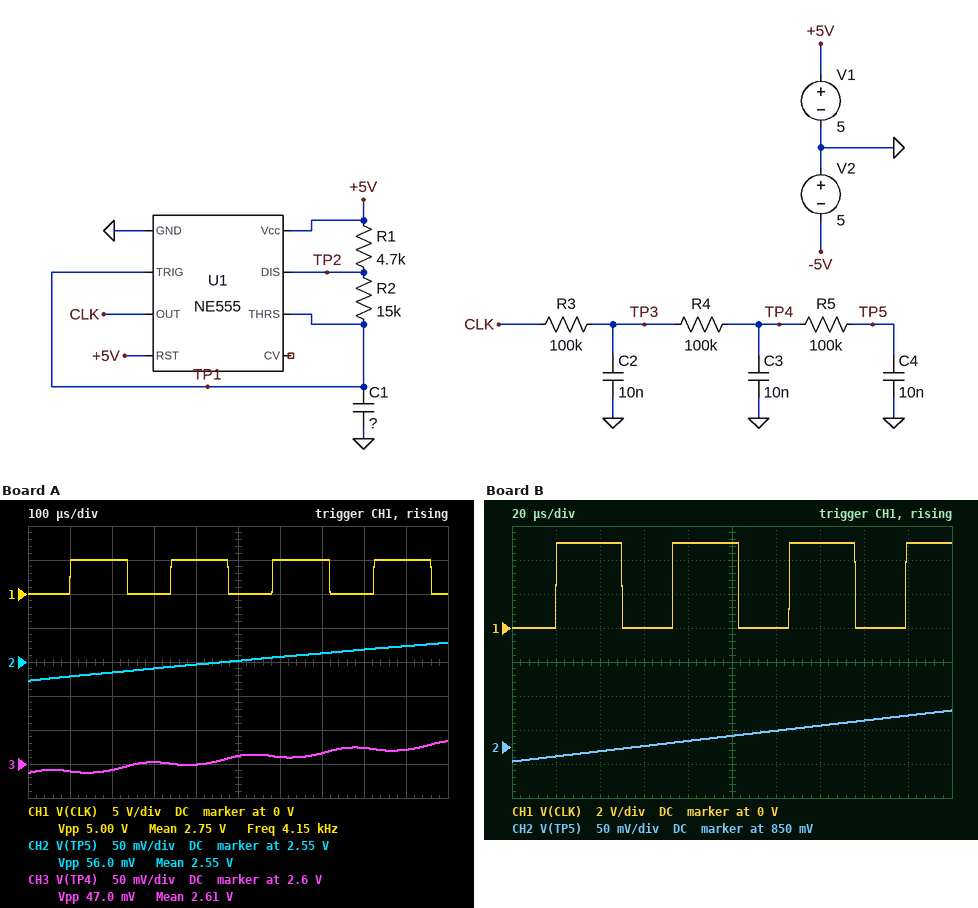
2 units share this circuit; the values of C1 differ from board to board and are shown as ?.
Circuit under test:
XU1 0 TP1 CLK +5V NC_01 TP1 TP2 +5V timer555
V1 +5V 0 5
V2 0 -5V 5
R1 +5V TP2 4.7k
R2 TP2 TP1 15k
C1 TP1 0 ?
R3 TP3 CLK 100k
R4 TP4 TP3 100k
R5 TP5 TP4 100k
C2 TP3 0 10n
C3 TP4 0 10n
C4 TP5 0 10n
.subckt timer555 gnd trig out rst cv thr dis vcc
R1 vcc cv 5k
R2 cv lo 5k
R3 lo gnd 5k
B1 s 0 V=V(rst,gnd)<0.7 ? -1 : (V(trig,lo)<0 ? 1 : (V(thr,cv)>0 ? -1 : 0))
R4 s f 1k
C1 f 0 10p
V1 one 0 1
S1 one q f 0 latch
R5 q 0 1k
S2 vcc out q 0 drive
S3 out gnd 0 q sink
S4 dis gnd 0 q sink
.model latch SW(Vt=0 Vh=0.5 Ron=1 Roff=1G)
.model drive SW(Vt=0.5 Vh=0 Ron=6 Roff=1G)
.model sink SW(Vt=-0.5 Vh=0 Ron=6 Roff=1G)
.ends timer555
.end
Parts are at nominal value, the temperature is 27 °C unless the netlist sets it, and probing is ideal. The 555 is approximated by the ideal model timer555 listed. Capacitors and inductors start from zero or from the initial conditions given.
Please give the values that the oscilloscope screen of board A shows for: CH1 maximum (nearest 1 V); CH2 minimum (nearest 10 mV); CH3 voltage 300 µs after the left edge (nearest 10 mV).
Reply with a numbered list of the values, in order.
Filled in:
1. 5 V
2. 2.52 V
3. 2.60 V
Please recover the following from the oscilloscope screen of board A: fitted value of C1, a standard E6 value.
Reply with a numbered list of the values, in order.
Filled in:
1. 10 nF
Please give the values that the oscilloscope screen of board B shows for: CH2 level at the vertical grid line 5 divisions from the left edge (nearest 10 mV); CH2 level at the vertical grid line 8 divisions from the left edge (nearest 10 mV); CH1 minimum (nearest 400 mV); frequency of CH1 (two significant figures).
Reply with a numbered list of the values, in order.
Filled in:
1. 870 mV
2. 890 mV
3. 0 V
4. 19 kHz
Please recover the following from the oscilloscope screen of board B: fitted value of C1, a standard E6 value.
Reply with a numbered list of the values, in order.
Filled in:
1. 2.2 nF
